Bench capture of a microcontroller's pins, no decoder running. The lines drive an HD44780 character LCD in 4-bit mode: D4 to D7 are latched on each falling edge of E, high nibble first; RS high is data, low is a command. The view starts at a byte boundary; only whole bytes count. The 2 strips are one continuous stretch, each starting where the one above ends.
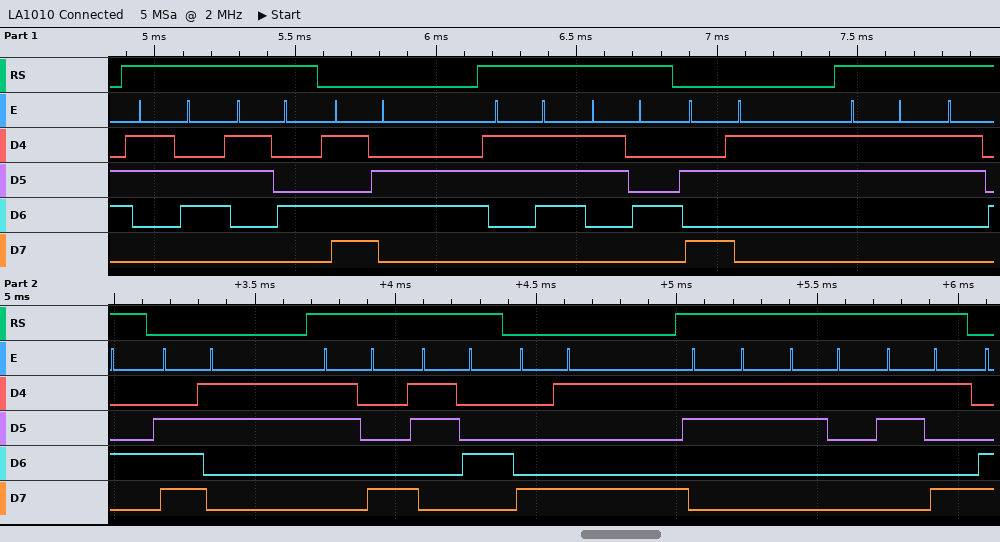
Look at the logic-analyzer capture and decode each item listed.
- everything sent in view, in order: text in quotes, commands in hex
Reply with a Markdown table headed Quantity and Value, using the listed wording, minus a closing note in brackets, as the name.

| Quantity | Value |
|---|---|
| everything sent in view, in order: text in quotes, commands in hex | "64" 0xD6 "74" 0xA3 "34" 0xE3 "84" 0x89 "319" |
